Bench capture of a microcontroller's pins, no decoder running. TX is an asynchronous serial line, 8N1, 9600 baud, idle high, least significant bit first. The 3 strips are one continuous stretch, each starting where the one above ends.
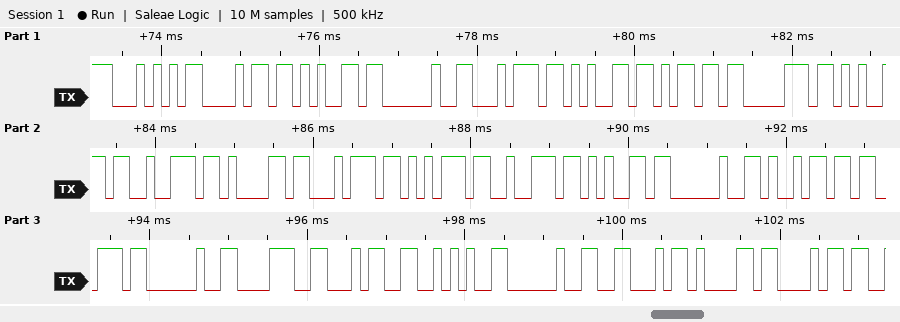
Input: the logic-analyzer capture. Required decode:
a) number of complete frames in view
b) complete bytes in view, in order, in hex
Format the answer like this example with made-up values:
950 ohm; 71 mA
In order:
26; 54 68 65 20 74 65 6D 70 65 72 61 74 75 72 65 20 69 73 20 38 34 2A 20 46 61 68
